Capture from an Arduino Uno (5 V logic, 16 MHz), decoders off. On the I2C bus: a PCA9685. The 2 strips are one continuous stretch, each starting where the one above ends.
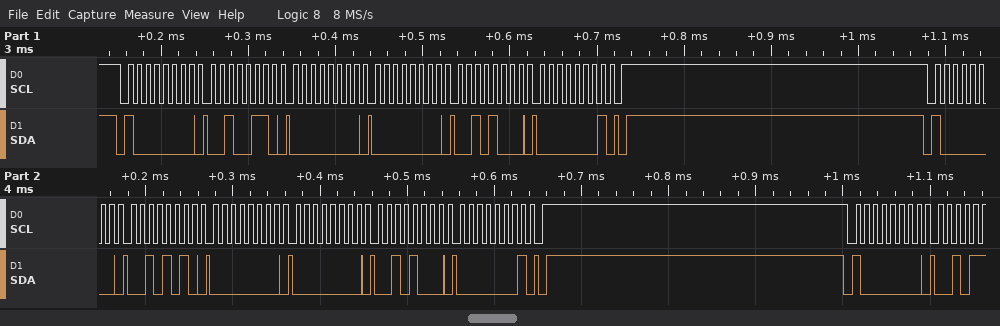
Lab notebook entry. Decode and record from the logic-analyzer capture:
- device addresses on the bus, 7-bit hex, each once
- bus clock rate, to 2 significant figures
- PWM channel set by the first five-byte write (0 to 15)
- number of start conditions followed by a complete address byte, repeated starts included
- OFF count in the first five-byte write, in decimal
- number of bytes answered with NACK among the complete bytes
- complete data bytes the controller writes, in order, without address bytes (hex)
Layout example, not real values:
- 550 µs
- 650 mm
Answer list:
- 0x40
- 100 kHz
- 8
- 3
- 296
- 0
- 26 00 00 28 01 2A 00 00 28 01
